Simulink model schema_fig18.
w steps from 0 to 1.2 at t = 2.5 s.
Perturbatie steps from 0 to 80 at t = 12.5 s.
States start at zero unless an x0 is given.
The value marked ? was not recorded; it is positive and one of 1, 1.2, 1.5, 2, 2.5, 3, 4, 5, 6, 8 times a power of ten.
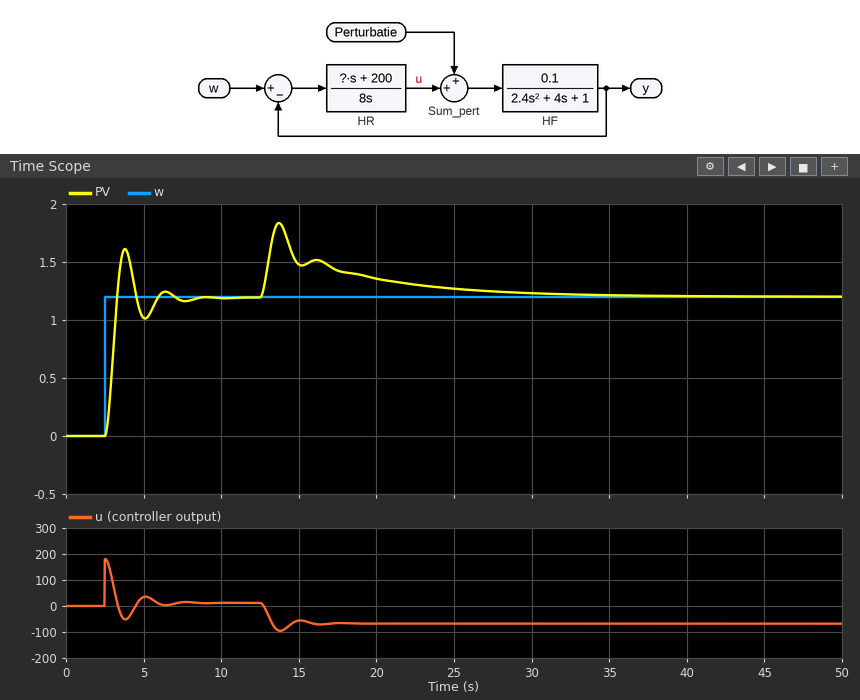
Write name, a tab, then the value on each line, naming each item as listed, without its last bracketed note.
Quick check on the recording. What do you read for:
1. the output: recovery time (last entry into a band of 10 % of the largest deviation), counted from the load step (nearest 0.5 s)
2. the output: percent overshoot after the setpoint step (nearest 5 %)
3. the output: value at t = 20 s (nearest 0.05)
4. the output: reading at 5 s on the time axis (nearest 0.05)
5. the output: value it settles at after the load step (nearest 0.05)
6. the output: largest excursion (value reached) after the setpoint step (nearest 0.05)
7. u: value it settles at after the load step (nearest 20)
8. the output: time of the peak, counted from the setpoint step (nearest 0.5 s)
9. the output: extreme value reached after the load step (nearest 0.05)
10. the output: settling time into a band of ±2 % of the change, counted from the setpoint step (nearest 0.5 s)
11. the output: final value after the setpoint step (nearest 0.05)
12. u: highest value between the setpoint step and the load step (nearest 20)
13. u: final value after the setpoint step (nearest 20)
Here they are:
the output: recovery time (last entry into a band of 10 % of the largest deviation), counted from the load step	13.0 s
the output: percent overshoot after the setpoint step	35 %
the output: value at t = 20 s	1.35
the output: reading at 5 s on the time axis	1.00
the output: value it settles at after the load step	1.20
the output: largest excursion (value reached) after the setpoint step	1.60
u: value it settles at after the load step	-60
the output: time of the peak, counted from the setpoint step	1.5 s
the output: extreme value reached after the load step	1.85
the output: settling time into a band of ±2 % of the change, counted from the setpoint step	5.5 s
the output: final value after the setpoint step	1.20
u: highest value between the setpoint step and the load step	180
u: final value after the setpoint step	20
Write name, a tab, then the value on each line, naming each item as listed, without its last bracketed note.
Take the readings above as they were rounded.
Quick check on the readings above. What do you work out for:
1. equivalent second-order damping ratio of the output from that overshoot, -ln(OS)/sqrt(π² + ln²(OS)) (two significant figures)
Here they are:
equivalent second-order damping ratio of the output from that overshoot, -ln(OS)/sqrt(π² + ln²(OS))	0.32
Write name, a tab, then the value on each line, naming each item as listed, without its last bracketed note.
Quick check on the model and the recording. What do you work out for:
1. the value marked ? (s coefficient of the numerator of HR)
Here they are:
the value marked ?	1200
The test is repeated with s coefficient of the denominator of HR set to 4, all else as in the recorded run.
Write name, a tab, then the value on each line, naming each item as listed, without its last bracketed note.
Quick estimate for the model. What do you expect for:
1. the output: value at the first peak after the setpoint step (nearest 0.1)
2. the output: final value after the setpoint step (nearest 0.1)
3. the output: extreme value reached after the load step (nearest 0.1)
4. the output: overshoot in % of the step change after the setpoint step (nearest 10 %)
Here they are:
the output: value at the first peak after the setpoint step	1.8
the output: final value after the setpoint step	1.2
the output: extreme value reached after the load step	1.6
the output: overshoot in % of the step change after the setpoint step	50 %
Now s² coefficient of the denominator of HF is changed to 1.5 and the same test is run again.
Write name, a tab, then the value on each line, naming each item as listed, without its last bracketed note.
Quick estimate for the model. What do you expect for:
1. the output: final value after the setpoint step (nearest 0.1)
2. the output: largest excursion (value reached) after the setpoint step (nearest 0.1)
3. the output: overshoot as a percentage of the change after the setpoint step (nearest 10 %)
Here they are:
the output: final value after the setpoint step	1.2
the output: largest excursion (value reached) after the setpoint step	1.5
the output: overshoot as a percentage of the change after the setpoint step	20 %
